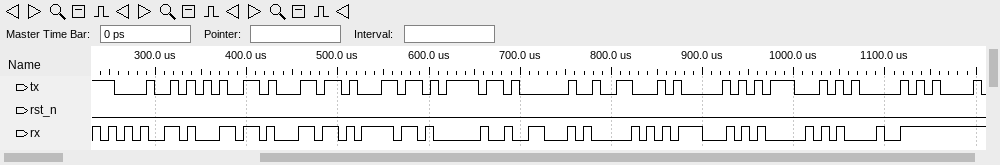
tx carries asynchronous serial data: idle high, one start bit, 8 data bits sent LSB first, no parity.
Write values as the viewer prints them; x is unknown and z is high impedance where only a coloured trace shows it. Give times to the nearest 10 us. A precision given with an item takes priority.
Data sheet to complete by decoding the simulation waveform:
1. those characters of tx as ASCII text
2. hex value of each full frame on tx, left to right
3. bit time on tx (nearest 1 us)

"Hello FPGA"
48, 65, 6C, 6C, 6F, 20, 46, 50, 47, 41
9 us
